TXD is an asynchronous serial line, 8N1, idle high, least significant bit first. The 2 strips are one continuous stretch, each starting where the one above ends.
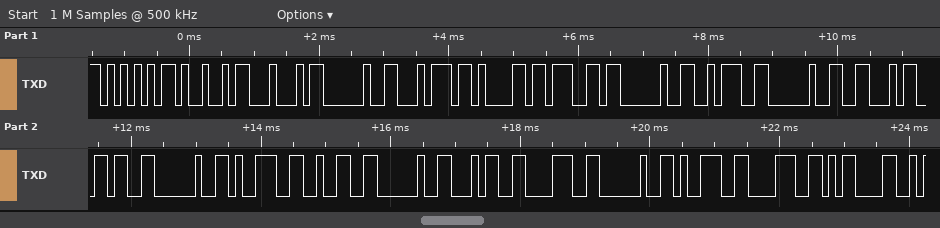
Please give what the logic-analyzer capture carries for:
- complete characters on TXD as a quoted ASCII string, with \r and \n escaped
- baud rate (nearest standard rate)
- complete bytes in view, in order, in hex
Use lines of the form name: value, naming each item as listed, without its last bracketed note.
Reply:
complete characters on TXD as a quoted ASCII string, with \r and \n escaped: "UID tag : F6 92 48 98\r"
baud rate: 9600 baud
complete bytes in view, in order, in hex: 55 49 44 20 74 61 67 20 3A 20 46 36 20 39 32 20 34 38 20 39 38 0D
